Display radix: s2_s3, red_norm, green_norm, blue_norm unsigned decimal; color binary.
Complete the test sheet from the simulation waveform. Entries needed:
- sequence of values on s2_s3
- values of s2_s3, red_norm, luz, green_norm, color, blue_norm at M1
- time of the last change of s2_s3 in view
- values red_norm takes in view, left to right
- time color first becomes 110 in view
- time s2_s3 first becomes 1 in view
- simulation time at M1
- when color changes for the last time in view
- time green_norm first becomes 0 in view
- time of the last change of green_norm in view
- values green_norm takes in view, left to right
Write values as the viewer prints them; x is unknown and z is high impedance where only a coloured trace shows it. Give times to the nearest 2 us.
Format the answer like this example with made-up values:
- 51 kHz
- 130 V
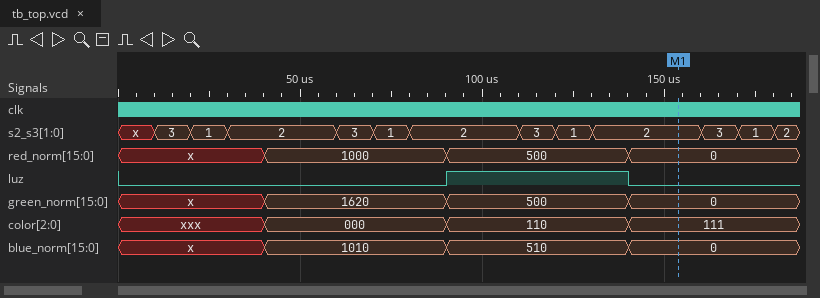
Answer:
- x, 3, 1, 2, 3, 1, 2, 3, 1, 2, 3, 1, 2
- s2_s3=2, red_norm=0, luz=0, green_norm=0, color=111, blue_norm=0
- 180 us
- x, 1000, 500, 0
- 90 us
- 20 us
- 154 us
- 140 us
- 140 us
- 140 us
- x, 1620, 500, 0
